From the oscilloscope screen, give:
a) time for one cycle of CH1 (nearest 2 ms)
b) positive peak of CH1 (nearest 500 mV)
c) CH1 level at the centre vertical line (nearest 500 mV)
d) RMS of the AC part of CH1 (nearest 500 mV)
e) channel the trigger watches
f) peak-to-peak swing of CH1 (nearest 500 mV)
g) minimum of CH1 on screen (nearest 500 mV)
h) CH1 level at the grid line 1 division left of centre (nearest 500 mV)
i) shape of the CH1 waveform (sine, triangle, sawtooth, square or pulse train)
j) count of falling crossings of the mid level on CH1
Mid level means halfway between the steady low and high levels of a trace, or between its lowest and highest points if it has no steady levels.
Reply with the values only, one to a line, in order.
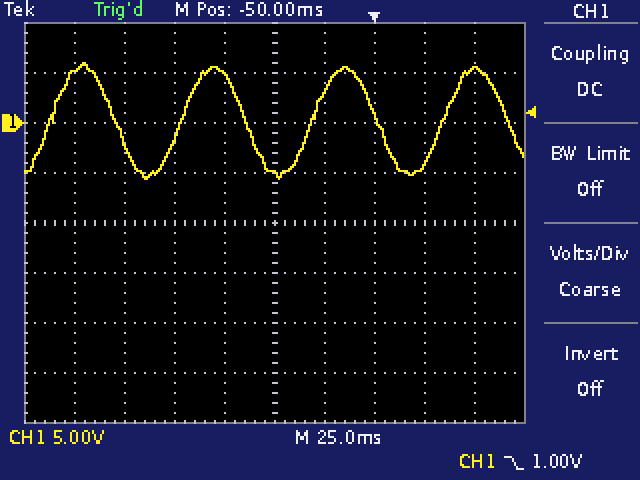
66 ms
6.0 V
-5.0 V
4.0 V
CH1
11.5 V
-5.5 V
5.0 V
sine
4
